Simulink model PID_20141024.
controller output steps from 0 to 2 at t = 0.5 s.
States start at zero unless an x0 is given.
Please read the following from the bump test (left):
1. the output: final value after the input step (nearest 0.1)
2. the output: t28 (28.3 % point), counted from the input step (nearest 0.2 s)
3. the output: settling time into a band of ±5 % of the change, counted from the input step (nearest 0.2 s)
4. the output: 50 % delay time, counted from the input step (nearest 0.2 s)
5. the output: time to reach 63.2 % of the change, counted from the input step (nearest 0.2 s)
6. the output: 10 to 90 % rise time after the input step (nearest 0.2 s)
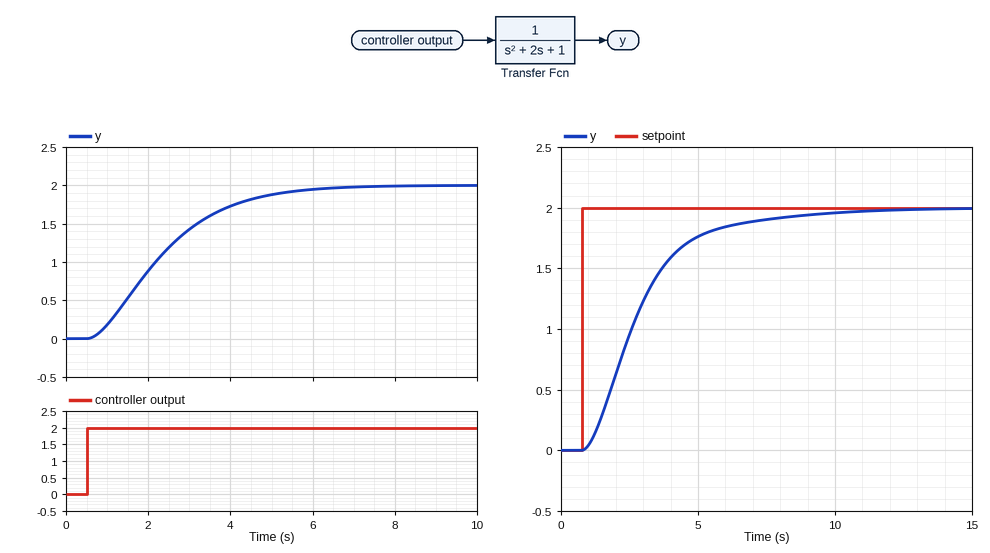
2.0
1.0 s
4.8 s
1.6 s
2.2 s
3.4 s
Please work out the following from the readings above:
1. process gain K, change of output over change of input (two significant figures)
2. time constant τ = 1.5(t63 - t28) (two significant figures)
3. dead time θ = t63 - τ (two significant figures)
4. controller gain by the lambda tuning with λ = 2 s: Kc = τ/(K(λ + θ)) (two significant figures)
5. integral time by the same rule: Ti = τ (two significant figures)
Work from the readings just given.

1.0
1.8 s
0.40 s
0.75
1.8 s
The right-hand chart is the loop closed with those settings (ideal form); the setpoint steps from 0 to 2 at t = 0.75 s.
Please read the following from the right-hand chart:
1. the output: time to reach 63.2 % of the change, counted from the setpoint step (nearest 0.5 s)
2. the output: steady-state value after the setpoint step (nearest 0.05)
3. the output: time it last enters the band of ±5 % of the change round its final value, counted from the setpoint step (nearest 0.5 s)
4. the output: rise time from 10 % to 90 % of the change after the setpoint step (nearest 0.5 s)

2.5 s
2.00
6.5 s
4.0 s
